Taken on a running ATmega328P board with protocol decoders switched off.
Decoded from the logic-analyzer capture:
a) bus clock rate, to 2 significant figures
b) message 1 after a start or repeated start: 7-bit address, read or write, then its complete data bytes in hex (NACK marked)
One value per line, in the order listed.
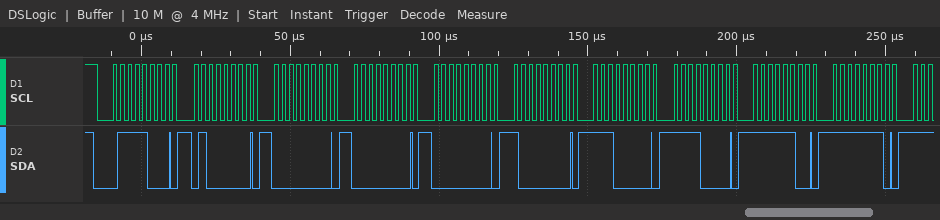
400 kHz
0x3C write: 40 00 00 00 80 E0 F0 FC FE
